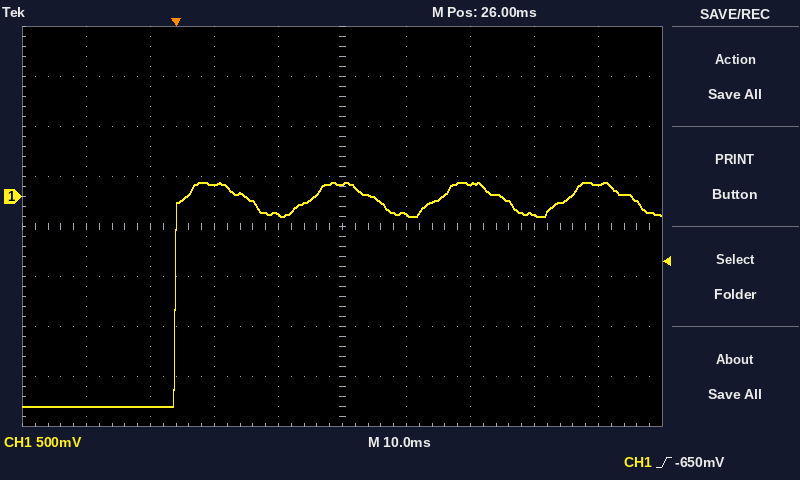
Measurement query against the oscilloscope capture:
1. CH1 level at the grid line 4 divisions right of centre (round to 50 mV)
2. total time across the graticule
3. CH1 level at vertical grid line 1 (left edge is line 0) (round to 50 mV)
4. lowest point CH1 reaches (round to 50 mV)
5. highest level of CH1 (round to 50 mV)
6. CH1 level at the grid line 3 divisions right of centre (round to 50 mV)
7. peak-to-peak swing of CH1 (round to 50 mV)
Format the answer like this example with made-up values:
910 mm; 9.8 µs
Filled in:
100 mV; 100 ms; -2.10 V; -2.10 V; 150 mV; -200 mV; 2.25 V
